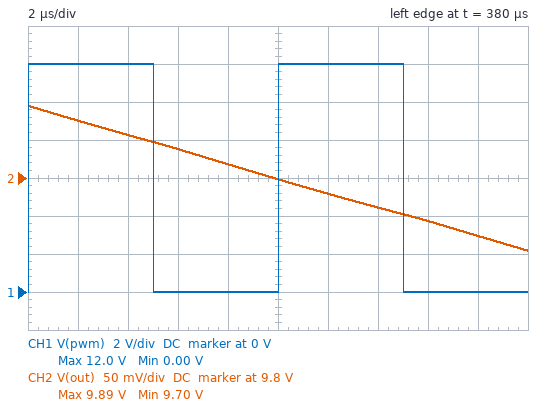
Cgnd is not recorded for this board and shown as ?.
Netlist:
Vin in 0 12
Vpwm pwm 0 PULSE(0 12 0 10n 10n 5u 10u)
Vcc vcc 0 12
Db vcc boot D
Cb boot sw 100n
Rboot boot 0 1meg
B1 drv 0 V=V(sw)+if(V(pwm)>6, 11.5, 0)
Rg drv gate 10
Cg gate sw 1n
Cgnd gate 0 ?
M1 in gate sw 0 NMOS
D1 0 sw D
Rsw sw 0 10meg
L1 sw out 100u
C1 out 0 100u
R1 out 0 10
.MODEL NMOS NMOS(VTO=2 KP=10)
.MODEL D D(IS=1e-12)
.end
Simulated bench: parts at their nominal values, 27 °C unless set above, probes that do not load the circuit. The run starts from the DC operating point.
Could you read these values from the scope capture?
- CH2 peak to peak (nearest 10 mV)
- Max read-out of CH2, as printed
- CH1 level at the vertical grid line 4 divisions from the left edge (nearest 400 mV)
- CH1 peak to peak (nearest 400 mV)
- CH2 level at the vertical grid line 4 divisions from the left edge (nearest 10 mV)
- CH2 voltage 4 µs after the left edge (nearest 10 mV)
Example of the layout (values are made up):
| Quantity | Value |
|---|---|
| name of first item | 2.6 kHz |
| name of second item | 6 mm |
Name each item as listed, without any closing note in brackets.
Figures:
| Quantity | Value |
|---|---|
| CH2 peak to peak | 190 mV |
| Max read-out of CH2, as printed | 9.89 V |
| CH1 level at the vertical grid line 4 divisions from the left edge | 0 V |
| CH1 peak to peak | 12.0 V |
| CH2 level at the vertical grid line 4 divisions from the left edge | 9.82 V |
| CH2 voltage 4 µs after the left edge | 9.86 V |
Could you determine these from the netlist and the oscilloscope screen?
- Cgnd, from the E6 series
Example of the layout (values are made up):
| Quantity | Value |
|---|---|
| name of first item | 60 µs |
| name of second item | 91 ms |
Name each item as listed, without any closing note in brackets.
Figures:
| Quantity | Value |
|---|---|
| Cgnd, from the E6 series | 680 pF |
